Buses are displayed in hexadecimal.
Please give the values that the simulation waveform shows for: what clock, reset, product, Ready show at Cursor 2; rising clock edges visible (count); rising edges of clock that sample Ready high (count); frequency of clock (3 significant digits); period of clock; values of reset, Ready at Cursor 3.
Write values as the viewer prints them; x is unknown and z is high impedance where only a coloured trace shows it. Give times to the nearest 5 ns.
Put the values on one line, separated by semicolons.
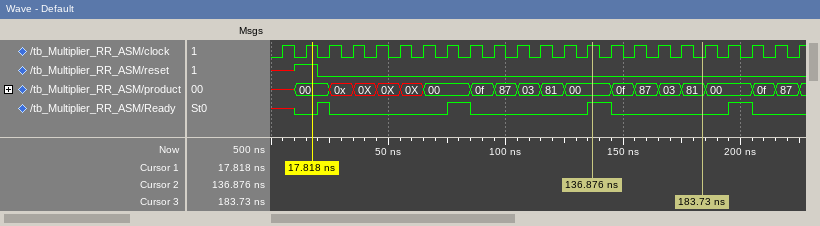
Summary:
clock=1, reset=0, product=00, Ready=1; 23; 4; 100 MHz; 10 ns; reset=0, Ready=0
